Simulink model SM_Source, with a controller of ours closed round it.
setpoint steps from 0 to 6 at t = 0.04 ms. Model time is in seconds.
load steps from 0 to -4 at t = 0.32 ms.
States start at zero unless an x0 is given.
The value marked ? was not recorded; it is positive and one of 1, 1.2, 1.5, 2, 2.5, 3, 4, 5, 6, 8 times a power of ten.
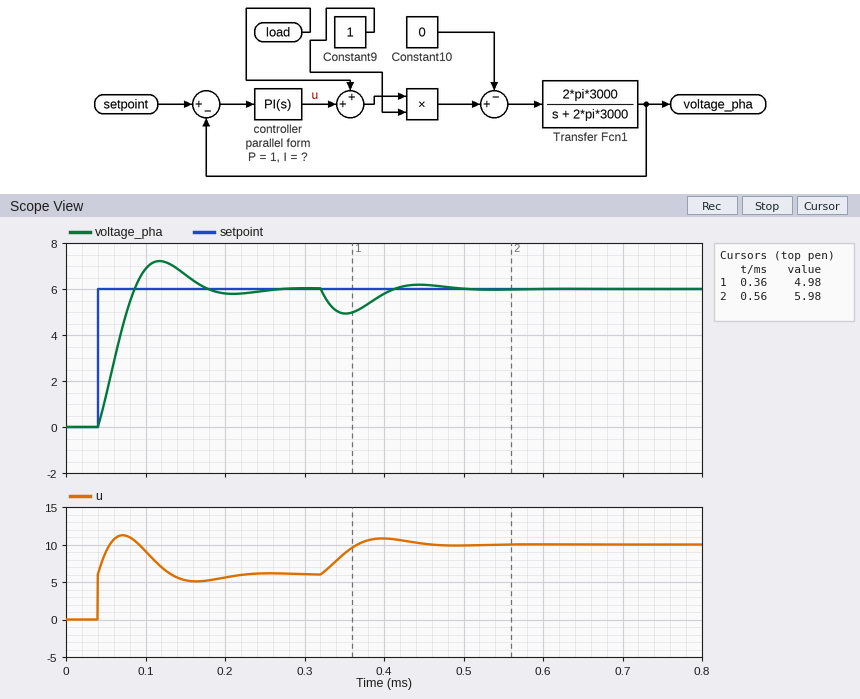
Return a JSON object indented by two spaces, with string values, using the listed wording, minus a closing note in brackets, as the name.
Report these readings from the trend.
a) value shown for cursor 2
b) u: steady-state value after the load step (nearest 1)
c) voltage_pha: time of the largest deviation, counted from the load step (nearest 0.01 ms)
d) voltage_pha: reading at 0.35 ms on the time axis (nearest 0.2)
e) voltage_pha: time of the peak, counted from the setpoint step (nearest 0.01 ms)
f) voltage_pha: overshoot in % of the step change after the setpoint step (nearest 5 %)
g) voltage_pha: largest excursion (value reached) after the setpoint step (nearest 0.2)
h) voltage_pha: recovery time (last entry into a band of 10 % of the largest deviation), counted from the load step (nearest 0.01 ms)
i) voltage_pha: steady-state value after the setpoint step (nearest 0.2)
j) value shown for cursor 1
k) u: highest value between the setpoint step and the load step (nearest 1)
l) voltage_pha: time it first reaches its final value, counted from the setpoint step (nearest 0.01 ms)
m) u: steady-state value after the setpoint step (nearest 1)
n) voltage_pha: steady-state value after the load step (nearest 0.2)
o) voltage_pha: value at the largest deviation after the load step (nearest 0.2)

{
  "value shown for cursor 2": "5.98",
  "u: steady-state value after the load step": "10",
  "voltage_pha: time of the largest deviation, counted from the load step": "0.03 ms",
  "voltage_pha: reading at 0.35 ms on the time axis": "5.0",
  "voltage_pha: time of the peak, counted from the setpoint step": "0.08 ms",
  "voltage_pha: overshoot in % of the step change after the setpoint step": "20 %",
  "voltage_pha: largest excursion (value reached) after the setpoint step": "7.2",
  "voltage_pha: recovery time (last entry into a band of 10 % of the largest deviation), counted from the load step": "0.15 ms",
  "voltage_pha: steady-state value after the setpoint step": "6.0",
  "value shown for cursor 1": "4.98",
  "u: highest value between the setpoint step and the load step": "11",
  "voltage_pha: time it first reaches its final value, counted from the setpoint step": "0.05 ms",
  "u: steady-state value after the setpoint step": "6",
  "voltage_pha: steady-state value after the load step": "6.0",
  "voltage_pha: value at the largest deviation after the load step": "5.0"
}
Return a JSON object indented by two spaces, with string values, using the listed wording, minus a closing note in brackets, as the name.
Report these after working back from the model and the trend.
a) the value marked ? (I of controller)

{
  "the value marked ?": "80000"
}
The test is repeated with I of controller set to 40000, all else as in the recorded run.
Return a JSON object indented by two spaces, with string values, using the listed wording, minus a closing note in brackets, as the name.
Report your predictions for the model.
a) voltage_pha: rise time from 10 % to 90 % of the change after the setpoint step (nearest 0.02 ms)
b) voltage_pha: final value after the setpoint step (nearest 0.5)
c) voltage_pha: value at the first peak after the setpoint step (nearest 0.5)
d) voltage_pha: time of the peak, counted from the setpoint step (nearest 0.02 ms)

{
  "voltage_pha: rise time from 10 % to 90 % of the change after the setpoint step": "0.06 ms",
  "voltage_pha: final value after the setpoint step": "6.0",
  "voltage_pha: value at the first peak after the setpoint step": "6.5",
  "voltage_pha: time of the peak, counted from the setpoint step": "0.12 ms"
}
